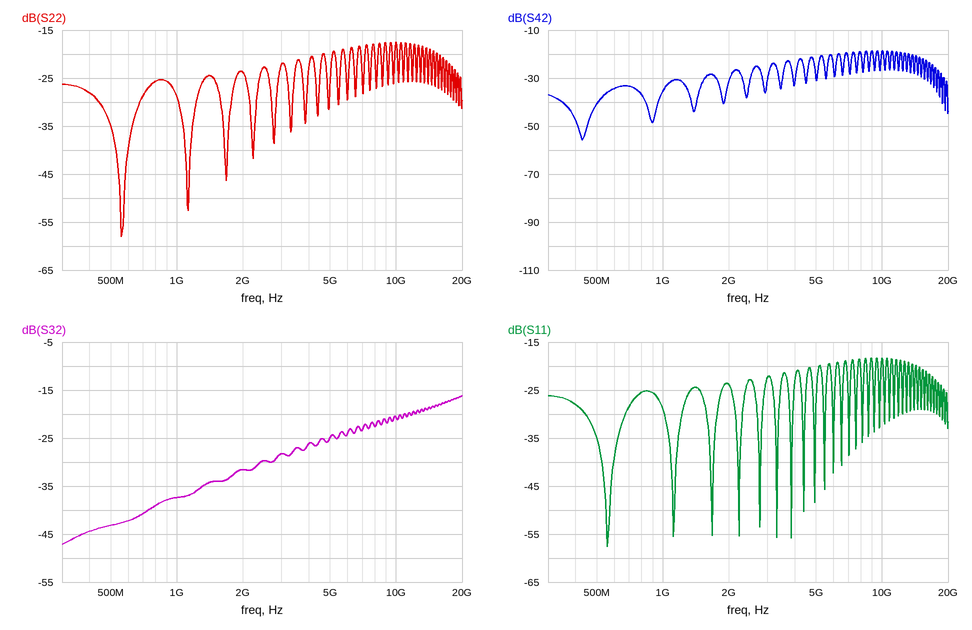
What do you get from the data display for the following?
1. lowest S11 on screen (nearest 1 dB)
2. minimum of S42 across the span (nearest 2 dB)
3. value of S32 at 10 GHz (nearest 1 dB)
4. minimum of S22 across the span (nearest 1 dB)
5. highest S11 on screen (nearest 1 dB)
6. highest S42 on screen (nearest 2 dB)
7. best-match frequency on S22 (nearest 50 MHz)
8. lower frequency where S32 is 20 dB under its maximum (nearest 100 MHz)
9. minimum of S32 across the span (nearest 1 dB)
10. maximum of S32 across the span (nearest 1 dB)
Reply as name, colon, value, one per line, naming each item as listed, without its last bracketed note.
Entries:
lowest S11 on screen: -58 dB
minimum of S42 across the span: -56 dB
value of S32 at 10 GHz: -21 dB
minimum of S22 across the span: -58 dB
highest S11 on screen: -18 dB
highest S42 on screen: -18 dB
best-match frequency on S22: 550 MHz
lower frequency where S32 is 20 dB under its maximum: 1.2 GHz
minimum of S32 across the span: -47 dB
maximum of S32 across the span: -16 dB
